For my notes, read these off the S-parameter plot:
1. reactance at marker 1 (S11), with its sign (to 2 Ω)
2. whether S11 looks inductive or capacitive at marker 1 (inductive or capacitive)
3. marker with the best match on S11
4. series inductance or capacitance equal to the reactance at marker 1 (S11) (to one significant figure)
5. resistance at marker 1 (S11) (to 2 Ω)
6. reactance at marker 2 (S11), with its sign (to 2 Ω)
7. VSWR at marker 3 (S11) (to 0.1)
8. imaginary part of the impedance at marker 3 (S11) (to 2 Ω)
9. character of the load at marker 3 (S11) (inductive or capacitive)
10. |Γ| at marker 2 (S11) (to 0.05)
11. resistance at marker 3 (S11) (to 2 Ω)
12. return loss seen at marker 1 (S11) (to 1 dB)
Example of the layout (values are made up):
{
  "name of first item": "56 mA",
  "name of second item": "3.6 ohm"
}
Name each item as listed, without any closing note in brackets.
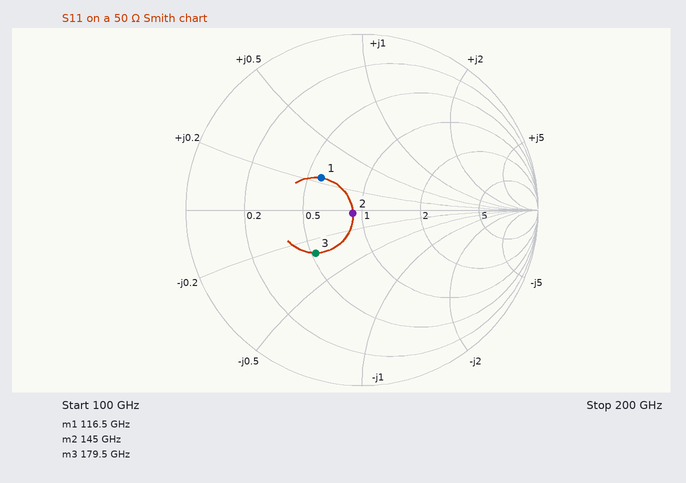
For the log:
{
  "reactance at marker 1 (S11), with its sign": "+12 Ω",
  "whether S11 looks inductive or capacitive at marker 1": "inductive",
  "marker with the best match on S11": "marker 2",
  "series inductance or capacitance equal to the reactance at marker 1 (S11)": "20 pH",
  "resistance at marker 1 (S11)": "30 Ω",
  "reactance at marker 2 (S11), with its sign": "-2 Ω",
  "VSWR at marker 3 (S11)": "2.1",
  "imaginary part of the impedance at marker 3 (S11)": "-14 Ω",
  "character of the load at marker 3 (S11)": "capacitive",
  "|Γ| at marker 2 (S11)": "0.05",
  "resistance at marker 3 (S11)": "26 Ω",
  "return loss seen at marker 1 (S11)": "11 dB"
}
